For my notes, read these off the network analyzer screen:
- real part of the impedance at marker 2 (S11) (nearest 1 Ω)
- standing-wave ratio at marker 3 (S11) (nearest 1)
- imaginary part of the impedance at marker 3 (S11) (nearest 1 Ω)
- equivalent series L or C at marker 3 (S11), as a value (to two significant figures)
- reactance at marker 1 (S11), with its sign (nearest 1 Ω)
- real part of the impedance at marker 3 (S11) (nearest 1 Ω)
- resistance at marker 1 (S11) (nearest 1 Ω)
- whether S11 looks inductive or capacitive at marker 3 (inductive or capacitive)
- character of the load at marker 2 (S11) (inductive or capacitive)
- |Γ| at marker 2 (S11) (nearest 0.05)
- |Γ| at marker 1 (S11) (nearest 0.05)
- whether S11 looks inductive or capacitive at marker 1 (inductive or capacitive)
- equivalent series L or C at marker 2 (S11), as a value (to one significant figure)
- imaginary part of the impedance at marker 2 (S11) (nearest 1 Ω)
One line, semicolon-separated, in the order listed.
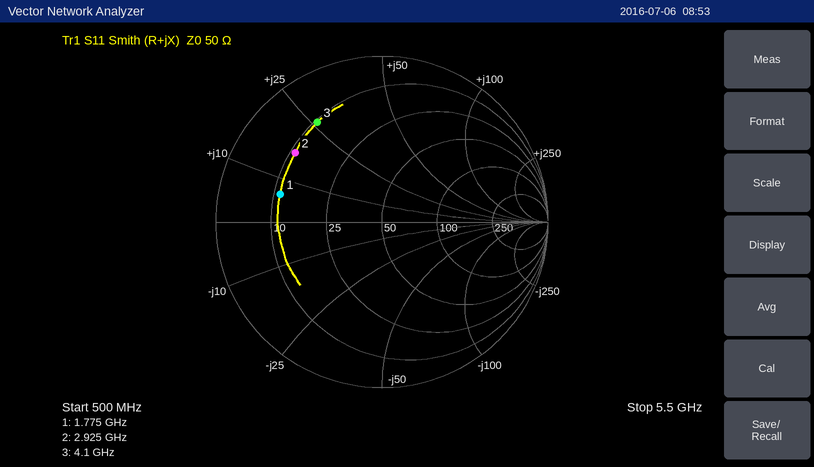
11 Ω; 6; +26 Ω; 1.0 nH; +6 Ω; 11 Ω; 11 Ω; inductive; inductive; 0.65; 0.65; inductive; 900 pH; +17 Ω
